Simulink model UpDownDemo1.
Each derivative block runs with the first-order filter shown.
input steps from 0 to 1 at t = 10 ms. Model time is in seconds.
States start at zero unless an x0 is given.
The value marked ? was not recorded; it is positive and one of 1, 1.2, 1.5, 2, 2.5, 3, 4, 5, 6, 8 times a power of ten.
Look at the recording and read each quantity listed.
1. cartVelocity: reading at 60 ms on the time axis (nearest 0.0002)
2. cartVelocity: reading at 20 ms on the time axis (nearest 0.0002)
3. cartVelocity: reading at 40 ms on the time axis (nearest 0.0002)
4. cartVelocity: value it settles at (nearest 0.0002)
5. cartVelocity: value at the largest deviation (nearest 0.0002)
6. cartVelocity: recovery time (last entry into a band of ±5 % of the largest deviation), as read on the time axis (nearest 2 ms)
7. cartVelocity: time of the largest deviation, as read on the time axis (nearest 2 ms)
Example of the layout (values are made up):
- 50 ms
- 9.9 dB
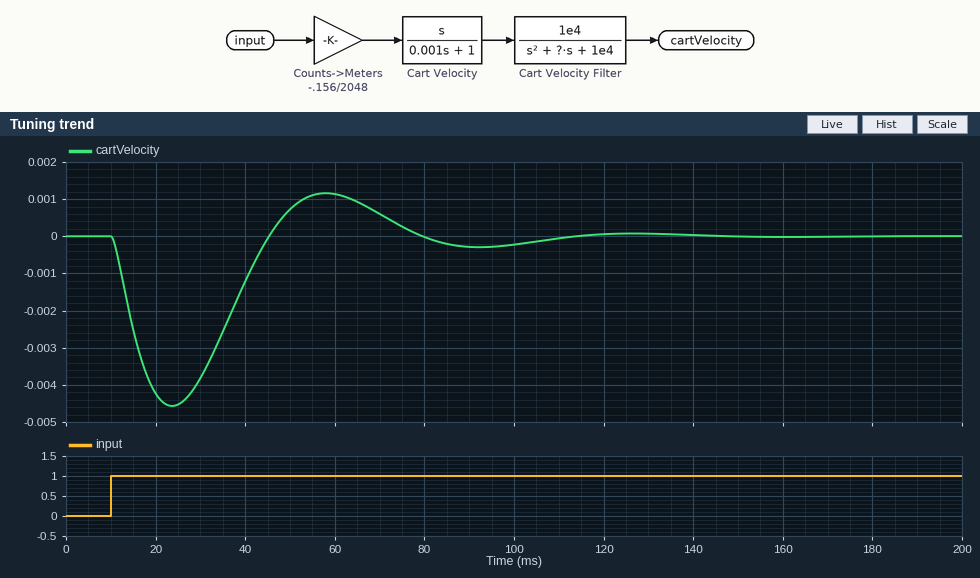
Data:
- 0.0012
- -0.0042
- -0.0012
- 0.0000
- -0.0046
- 100 ms
- 24 ms
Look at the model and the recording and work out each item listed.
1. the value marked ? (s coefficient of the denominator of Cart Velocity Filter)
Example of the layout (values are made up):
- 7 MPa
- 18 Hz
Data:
- 80
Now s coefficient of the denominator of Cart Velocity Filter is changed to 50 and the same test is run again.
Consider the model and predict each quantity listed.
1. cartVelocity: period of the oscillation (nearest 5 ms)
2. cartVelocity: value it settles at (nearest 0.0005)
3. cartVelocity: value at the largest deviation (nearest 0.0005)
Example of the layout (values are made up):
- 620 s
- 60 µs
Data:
- 65 ms
- 0.0000
- -0.0055
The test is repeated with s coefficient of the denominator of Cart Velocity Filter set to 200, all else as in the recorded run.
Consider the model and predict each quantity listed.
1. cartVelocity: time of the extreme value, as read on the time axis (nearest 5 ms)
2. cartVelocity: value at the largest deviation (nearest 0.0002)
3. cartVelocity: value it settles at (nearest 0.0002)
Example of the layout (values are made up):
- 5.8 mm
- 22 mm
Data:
- 20 ms
- -0.0028
- 0.0000
